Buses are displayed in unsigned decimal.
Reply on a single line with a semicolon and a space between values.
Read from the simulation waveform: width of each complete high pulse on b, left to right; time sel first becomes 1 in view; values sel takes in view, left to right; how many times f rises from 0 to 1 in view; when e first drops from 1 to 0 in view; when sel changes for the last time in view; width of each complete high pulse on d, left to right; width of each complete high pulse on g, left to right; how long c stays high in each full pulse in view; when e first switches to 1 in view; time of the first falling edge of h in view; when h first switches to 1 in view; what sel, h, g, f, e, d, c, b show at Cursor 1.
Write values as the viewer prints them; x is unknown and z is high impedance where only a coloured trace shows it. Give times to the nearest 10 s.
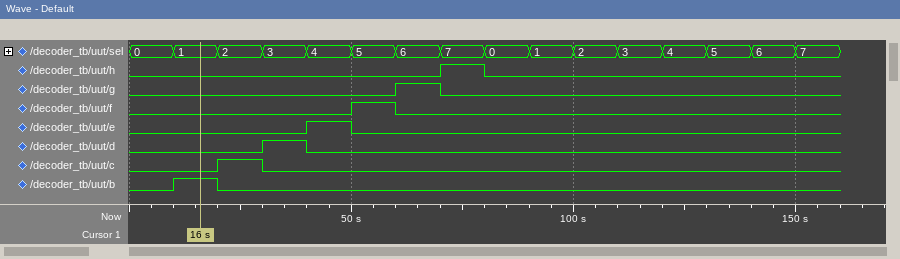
10 s; 10 s; 0, 1, 2, 3, 4, 5, 6, 7, 0, 1, 2, 3, 4, 5, 6, 7; 1; 50 s; 150 s; 10 s; 10 s; 10 s; 40 s; 80 s; 70 s; sel=1, h=0, g=0, f=0, e=0, d=0, c=0, b=1
